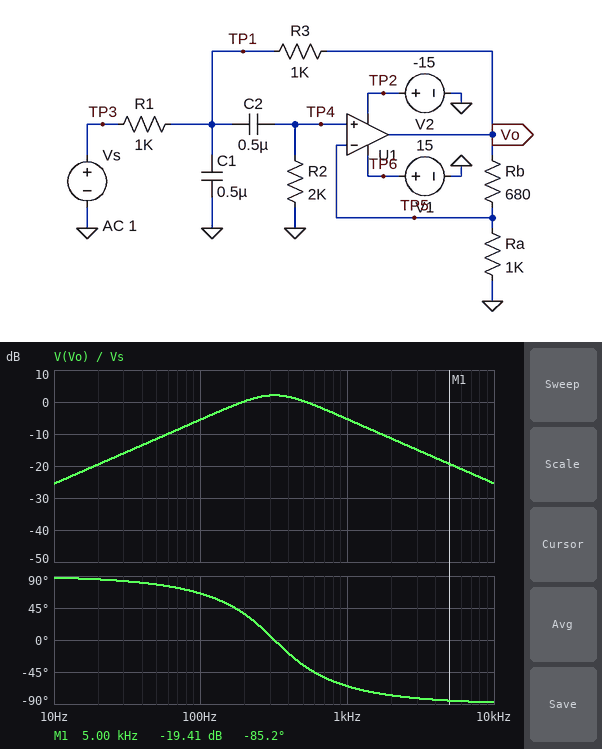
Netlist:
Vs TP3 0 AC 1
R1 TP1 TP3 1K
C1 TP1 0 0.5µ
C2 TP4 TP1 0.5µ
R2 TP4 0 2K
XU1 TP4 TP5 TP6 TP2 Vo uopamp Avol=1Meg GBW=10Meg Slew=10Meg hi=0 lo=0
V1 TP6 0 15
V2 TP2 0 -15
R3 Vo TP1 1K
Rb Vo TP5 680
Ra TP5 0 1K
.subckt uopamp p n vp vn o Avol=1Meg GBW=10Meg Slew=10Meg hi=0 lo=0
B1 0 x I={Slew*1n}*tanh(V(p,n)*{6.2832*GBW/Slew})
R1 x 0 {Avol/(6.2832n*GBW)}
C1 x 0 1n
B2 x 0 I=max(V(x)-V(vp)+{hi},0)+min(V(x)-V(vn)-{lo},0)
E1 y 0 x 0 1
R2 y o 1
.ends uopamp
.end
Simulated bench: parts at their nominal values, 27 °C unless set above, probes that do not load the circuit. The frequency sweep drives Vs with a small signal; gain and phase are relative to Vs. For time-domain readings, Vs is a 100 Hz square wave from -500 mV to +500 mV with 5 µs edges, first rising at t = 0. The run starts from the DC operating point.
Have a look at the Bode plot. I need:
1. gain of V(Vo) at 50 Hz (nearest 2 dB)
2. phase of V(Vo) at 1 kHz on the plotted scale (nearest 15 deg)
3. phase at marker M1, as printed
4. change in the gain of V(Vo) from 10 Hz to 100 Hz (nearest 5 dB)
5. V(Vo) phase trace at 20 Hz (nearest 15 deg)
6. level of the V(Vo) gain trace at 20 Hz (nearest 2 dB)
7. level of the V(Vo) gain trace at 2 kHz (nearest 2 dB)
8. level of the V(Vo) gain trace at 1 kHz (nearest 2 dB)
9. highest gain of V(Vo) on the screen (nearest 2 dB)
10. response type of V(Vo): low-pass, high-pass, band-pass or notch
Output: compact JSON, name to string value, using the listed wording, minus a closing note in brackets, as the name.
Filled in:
{"gain of V(Vo) at 50 Hz": "-12 dB", "phase of V(Vo) at 1 kHz on the plotted scale": "-60 deg", "phase at marker M1, as printed": "-85.2 deg", "change in the gain of V(Vo) from 10 Hz to 100 Hz": "20 dB", "V(Vo) phase trace at 20 Hz": "90 deg", "level of the V(Vo) gain trace at 20 Hz": "-20 dB", "level of the V(Vo) gain trace at 2 kHz": "-12 dB", "level of the V(Vo) gain trace at 1 kHz": "-6 dB", "highest gain of V(Vo) on the screen": "2 dB", "response type of V(Vo): low-pass, high-pass, band-pass or notch": "band-pass"}
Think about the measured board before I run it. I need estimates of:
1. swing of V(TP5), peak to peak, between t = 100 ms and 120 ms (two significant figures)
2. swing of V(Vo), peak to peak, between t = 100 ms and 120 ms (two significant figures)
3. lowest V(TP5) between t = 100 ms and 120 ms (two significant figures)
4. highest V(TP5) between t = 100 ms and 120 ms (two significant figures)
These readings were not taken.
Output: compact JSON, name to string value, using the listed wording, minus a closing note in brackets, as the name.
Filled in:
{"swing of V(TP5), peak to peak, between t = 100 ms and 120 ms": "950 mV", "swing of V(Vo), peak to peak, between t = 100 ms and 120 ms": "1.6 V", "lowest V(TP5) between t = 100 ms and 120 ms": "-470 mV", "highest V(TP5) between t = 100 ms and 120 ms": "470 mV"}
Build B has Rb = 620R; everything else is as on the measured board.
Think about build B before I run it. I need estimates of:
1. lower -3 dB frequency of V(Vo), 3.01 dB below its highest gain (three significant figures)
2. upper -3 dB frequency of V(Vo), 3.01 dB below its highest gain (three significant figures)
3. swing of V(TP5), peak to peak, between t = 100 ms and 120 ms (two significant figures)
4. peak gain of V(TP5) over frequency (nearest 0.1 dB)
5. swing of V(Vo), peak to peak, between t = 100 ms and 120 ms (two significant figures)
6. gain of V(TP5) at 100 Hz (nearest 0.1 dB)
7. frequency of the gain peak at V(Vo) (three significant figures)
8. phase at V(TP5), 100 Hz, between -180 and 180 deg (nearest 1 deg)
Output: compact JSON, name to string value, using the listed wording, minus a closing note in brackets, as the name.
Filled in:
{"lower -3 dB frequency of V(Vo), 3.01 dB below its highest gain": "167 Hz", "upper -3 dB frequency of V(Vo), 3.01 dB below its highest gain": "606 Hz", "swing of V(TP5), peak to peak, between t = 100 ms and 120 ms": "920 mV", "peak gain of V(TP5) over frequency": "-2.8 dB", "swing of V(Vo), peak to peak, between t = 100 ms and 120 ms": "1.5 V", "gain of V(TP5) at 100 Hz": "-10.1 dB", "frequency of the gain peak at V(Vo)": "318 Hz", "phase at V(TP5), 100 Hz, between -180 and 180 deg": "64 deg"}
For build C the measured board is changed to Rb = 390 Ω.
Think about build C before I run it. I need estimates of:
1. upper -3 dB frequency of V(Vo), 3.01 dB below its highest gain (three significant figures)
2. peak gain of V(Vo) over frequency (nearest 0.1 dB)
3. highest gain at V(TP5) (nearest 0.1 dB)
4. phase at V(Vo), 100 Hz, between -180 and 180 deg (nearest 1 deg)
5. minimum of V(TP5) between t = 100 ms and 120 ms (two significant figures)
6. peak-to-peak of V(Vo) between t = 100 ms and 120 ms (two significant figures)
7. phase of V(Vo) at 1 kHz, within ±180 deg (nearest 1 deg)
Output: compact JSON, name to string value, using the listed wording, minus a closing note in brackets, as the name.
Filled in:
{"upper -3 dB frequency of V(Vo), 3.01 dB below its highest gain": "665 Hz", "peak gain of V(Vo) over frequency": "-1.3 dB", "highest gain at V(TP5)": "-4.1 dB", "phase at V(Vo), 100 Hz, between -180 and 180 deg": "61 deg", "minimum of V(TP5) between t = 100 ms and 120 ms": "-420 mV", "peak-to-peak of V(Vo) between t = 100 ms and 120 ms": "1.2 V", "phase of V(Vo) at 1 kHz, within ±180 deg": "-60 deg"}
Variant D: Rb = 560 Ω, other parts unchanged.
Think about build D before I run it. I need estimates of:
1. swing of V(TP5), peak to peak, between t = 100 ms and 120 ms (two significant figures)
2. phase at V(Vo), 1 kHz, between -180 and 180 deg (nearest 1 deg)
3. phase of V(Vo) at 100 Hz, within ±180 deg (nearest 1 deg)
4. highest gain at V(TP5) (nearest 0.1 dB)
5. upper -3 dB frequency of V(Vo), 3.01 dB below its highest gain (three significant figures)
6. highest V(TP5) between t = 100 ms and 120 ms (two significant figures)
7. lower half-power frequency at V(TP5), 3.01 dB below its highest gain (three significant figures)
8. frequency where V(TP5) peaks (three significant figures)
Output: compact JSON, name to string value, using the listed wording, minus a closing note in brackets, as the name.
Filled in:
{"swing of V(TP5), peak to peak, between t = 100 ms and 120 ms": "900 mV", "phase at V(Vo), 1 kHz, between -180 and 180 deg": "-63 deg", "phase of V(Vo) at 100 Hz, within ±180 deg": "63 deg", "highest gain at V(TP5)": "-3.2 dB", "upper -3 dB frequency of V(Vo), 3.01 dB below its highest gain": "621 Hz", "highest V(TP5) between t = 100 ms and 120 ms": "450 mV", "lower half-power frequency at V(TP5), 3.01 dB below its highest gain": "163 Hz", "frequency where V(TP5) peaks": "318 Hz"}
